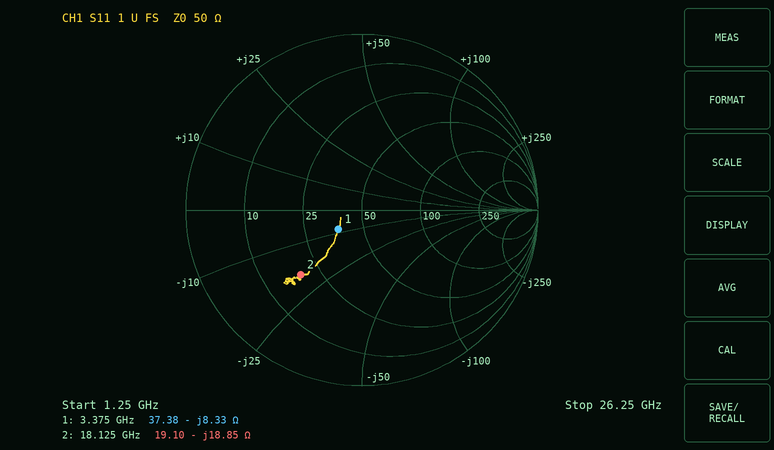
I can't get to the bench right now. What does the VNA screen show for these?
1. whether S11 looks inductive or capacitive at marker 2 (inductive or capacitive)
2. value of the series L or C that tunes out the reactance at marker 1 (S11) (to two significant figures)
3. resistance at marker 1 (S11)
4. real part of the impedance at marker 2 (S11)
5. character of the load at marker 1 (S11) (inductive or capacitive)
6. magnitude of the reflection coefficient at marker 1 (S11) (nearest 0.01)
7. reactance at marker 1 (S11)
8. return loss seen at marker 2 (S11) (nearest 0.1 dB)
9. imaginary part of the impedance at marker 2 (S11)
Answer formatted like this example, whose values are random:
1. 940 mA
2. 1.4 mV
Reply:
1. capacitive
2. 390 pH
3. 37.38 Ω
4. 19.10 Ω
5. capacitive
6. 0.17
7. -8.33 Ω
8. 5.9 dB
9. -18.85 Ω
